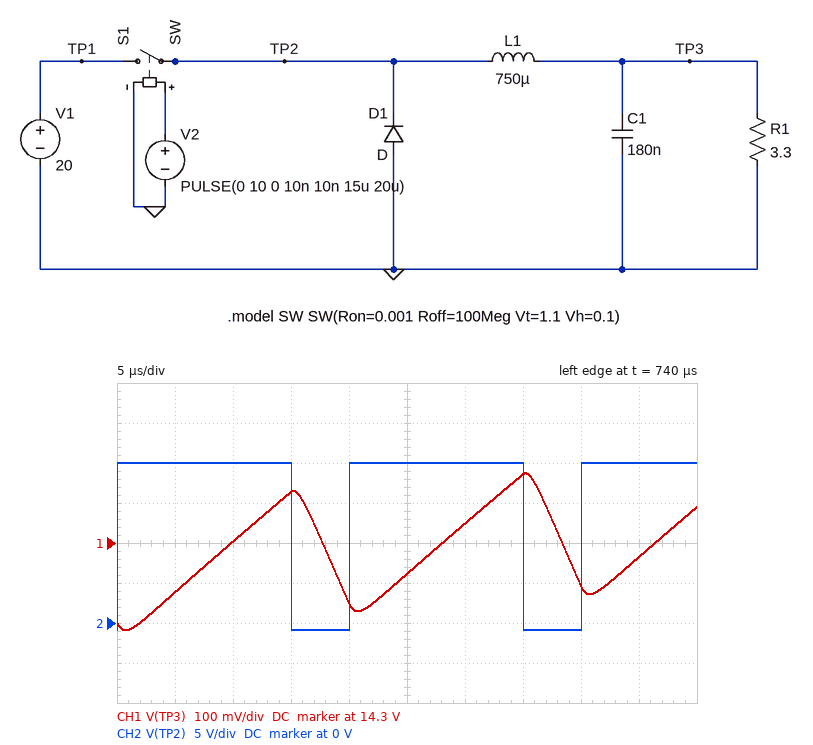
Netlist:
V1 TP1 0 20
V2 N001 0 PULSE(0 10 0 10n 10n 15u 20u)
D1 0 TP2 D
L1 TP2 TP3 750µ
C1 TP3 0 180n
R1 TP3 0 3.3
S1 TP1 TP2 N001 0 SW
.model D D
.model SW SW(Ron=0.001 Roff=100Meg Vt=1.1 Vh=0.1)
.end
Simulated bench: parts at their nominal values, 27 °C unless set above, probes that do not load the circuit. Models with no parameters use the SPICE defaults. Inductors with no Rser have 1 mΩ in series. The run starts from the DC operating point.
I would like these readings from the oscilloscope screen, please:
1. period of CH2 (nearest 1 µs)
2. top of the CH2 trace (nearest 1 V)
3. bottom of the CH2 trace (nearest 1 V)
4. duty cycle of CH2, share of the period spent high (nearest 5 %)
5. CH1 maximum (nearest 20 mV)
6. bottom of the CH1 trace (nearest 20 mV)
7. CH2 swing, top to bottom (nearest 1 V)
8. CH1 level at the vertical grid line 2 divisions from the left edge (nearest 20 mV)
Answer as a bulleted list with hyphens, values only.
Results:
- 20 µs
- 20 V
- -1 V
- 75 %
- 14.48 V
- 14.08 V
- 21 V
- 14.30 V
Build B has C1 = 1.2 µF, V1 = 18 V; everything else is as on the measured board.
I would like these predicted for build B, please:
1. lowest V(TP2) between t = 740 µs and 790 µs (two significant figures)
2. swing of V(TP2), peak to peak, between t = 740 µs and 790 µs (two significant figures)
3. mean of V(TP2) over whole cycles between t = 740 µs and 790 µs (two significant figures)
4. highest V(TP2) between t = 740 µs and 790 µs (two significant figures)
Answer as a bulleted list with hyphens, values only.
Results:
- -870 mV
- 19 V
- 13 V
- 18 V
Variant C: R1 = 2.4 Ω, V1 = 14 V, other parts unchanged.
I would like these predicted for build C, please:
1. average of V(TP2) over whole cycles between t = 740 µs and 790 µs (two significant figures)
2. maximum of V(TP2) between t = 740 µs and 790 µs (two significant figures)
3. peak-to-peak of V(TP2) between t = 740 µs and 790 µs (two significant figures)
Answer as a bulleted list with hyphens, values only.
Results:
- 10 V
- 14 V
- 15 V
